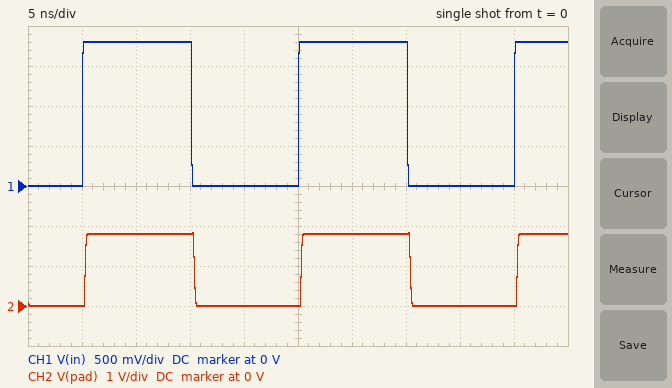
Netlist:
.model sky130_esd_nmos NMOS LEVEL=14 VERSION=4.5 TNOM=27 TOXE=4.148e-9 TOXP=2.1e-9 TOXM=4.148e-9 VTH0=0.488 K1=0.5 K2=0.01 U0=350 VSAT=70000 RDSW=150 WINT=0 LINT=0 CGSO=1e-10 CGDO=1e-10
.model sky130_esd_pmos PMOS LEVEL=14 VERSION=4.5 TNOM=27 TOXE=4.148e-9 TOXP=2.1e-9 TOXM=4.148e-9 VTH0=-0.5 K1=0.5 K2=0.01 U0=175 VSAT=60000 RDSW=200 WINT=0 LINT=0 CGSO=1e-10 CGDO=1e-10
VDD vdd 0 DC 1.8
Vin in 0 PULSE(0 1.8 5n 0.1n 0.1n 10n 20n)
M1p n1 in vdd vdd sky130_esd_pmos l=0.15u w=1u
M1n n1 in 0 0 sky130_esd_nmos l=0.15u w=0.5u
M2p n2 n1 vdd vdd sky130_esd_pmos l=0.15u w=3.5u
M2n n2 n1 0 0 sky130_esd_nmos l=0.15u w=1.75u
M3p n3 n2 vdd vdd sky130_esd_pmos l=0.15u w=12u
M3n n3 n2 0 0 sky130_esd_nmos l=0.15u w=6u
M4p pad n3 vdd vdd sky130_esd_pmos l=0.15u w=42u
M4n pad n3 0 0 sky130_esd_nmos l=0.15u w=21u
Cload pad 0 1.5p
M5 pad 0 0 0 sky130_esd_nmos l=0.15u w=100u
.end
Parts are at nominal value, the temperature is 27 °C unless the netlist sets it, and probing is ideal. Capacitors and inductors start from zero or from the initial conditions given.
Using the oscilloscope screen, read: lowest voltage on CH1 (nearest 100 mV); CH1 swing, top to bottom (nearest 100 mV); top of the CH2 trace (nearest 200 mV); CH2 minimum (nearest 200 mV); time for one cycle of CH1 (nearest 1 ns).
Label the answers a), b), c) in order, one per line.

a) 0 V
b) 1.8 V
c) 1.8 V
d) 0 V
e) 20 ns
